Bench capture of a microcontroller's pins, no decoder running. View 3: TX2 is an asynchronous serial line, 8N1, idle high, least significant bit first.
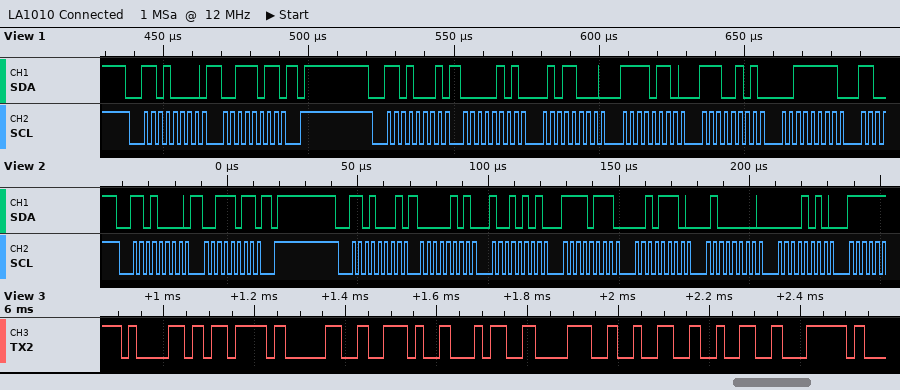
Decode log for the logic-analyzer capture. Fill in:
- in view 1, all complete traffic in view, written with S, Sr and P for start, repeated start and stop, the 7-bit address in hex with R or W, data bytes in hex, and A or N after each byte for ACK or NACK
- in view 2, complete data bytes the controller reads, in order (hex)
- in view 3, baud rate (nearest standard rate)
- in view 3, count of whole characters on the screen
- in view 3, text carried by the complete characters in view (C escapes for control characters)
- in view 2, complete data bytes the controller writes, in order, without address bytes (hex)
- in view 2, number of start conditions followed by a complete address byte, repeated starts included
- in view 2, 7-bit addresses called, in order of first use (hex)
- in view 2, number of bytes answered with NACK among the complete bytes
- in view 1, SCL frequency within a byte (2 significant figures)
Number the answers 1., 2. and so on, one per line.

1. S 68W A 3B A P S 68R A 05 A 58 A F6 A E5 A 3F A
2. 05 95 F7 2E 40 0A
3. 57600 baud
4. 9
5. "a{0.4822|"
6. 3B
7. 2
8. 0x68
9. 0
10. 400 kHz
